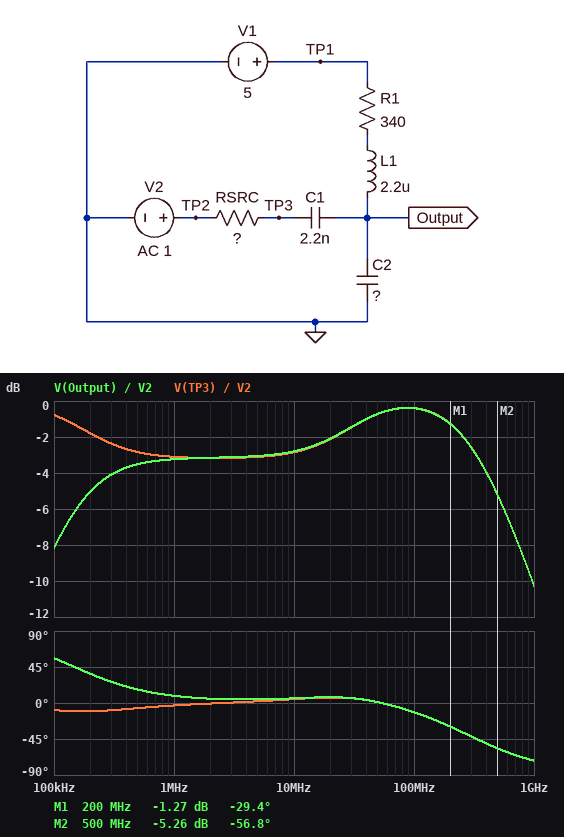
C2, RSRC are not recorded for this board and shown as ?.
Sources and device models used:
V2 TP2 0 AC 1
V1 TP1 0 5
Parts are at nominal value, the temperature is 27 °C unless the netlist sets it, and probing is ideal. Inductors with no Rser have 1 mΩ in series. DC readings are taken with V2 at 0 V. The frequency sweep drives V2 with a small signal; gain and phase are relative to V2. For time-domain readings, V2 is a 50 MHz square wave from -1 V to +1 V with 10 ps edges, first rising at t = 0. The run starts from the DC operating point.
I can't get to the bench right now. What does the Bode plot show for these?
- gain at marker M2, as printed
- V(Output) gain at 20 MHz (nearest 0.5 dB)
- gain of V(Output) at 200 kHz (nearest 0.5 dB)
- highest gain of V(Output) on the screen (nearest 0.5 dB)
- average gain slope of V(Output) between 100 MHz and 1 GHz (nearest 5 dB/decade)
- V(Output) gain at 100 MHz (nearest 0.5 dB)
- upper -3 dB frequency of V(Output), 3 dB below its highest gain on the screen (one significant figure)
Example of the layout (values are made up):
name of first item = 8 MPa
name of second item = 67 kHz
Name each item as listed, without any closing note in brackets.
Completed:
gain at marker M2, as printed = -5.26 dB
V(Output) gain at 20 MHz = -2.0 dB
gain of V(Output) at 200 kHz = -5.0 dB
highest gain of V(Output) on the screen = -0.5 dB
average gain slope of V(Output) between 100 MHz and 1 GHz = -10 dB/decade
V(Output) gain at 100 MHz = -0.5 dB
upper -3 dB frequency of V(Output), 3 dB below its highest gain on the screen = 400 MHz
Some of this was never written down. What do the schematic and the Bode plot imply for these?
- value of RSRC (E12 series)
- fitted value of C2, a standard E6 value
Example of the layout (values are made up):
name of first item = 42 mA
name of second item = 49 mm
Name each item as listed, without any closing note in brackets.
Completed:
value of RSRC = 150 Ω
fitted value of C2, a standard E6 value = 3.3 pF
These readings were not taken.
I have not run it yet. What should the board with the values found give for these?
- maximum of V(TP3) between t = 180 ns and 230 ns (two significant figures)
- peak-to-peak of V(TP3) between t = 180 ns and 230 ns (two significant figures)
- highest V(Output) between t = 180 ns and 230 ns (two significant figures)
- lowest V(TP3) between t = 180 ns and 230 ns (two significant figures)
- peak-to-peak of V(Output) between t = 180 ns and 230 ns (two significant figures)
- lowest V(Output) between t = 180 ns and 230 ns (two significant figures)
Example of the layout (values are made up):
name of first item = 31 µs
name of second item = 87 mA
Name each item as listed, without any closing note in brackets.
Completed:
maximum of V(TP3) between t = 180 ns and 230 ns = 850 mV
peak-to-peak of V(TP3) between t = 180 ns and 230 ns = 2.2 V
highest V(Output) between t = 180 ns and 230 ns = 6.7 V
lowest V(TP3) between t = 180 ns and 230 ns = -1.4 V
peak-to-peak of V(Output) between t = 180 ns and 230 ns = 2.2 V
lowest V(Output) between t = 180 ns and 230 ns = 4.5 V
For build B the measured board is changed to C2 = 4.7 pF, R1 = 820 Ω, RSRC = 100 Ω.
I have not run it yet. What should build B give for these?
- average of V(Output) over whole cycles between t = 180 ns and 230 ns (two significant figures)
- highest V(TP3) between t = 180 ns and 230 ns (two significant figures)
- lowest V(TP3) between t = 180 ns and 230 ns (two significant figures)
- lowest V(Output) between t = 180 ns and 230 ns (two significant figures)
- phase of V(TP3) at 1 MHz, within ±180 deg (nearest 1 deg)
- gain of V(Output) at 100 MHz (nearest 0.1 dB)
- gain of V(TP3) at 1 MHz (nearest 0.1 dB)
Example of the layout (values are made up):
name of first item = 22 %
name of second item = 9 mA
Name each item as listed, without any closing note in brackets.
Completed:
average of V(Output) over whole cycles between t = 180 ns and 230 ns = 5.8 V
highest V(TP3) between t = 180 ns and 230 ns = 900 mV
lowest V(TP3) between t = 180 ns and 230 ns = -1.1 V
lowest V(Output) between t = 180 ns and 230 ns = 4.8 V
phase of V(TP3) at 1 MHz, within ±180 deg = -1 deg
gain of V(Output) at 100 MHz = -0.5 dB
gain of V(TP3) at 1 MHz = -1.0 dB
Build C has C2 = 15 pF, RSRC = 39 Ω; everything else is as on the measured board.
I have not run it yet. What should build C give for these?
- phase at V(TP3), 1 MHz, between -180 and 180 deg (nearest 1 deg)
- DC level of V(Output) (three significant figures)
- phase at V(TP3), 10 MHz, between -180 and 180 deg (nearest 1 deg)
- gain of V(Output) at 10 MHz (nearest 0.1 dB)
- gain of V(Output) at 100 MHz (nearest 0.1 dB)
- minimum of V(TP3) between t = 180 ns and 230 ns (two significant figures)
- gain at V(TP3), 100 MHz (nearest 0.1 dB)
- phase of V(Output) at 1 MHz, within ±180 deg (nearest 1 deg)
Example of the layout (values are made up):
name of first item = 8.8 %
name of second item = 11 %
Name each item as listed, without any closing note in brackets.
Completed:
phase at V(TP3), 1 MHz, between -180 and 180 deg = -1 deg
DC level of V(Output) = 5.00 V
phase at V(TP3), 10 MHz, between -180 and 180 deg = 0 deg
gain of V(Output) at 10 MHz = -0.8 dB
gain of V(Output) at 100 MHz = -0.6 dB
minimum of V(TP3) between t = 180 ns and 230 ns = -1.1 V
gain at V(TP3), 100 MHz = -0.5 dB
phase of V(Output) at 1 MHz, within ±180 deg = 11 deg
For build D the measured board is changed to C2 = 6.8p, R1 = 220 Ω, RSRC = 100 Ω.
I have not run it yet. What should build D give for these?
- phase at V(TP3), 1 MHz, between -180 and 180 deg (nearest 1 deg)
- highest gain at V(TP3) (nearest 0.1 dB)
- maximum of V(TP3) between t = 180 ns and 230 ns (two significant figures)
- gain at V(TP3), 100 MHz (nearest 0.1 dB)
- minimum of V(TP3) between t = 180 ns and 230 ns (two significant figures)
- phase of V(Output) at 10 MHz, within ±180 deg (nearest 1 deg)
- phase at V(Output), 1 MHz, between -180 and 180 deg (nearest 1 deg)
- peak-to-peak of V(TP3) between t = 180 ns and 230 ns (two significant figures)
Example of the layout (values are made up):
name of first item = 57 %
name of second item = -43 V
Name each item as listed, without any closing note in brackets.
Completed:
phase at V(TP3), 1 MHz, between -180 and 180 deg = -5 deg
highest gain at V(TP3) = 0 dB
maximum of V(TP3) between t = 180 ns and 230 ns = 840 mV
gain at V(TP3), 100 MHz = -0.6 dB
minimum of V(TP3) between t = 180 ns and 230 ns = -1.3 V
phase of V(Output) at 10 MHz, within ±180 deg = 8 deg
phase at V(Output), 1 MHz, between -180 and 180 deg = 14 deg
peak-to-peak of V(TP3) between t = 180 ns and 230 ns = 2.1 V
